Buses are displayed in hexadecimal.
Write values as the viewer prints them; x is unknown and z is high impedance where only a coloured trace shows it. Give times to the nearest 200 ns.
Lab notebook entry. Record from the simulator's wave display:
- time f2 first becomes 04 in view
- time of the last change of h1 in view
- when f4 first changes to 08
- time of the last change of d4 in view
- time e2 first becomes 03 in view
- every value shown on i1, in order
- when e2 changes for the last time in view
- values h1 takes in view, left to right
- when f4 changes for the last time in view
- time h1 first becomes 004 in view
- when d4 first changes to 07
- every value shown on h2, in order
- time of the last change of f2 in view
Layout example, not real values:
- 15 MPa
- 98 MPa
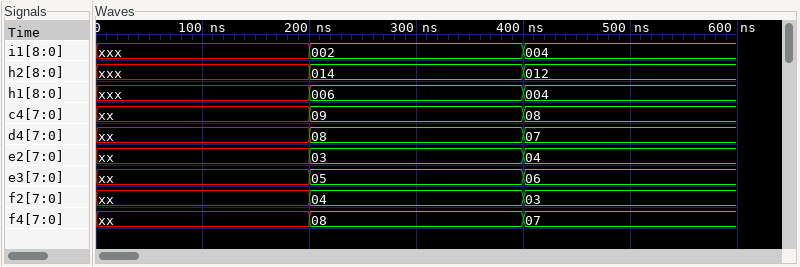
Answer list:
- 200 ns
- 400 ns
- 200 ns
- 400 ns
- 200 ns
- xxx, 002, 004
- 400 ns
- xxx, 006, 004
- 400 ns
- 400 ns
- 400 ns
- xxx, 014, 012
- 400 ns
